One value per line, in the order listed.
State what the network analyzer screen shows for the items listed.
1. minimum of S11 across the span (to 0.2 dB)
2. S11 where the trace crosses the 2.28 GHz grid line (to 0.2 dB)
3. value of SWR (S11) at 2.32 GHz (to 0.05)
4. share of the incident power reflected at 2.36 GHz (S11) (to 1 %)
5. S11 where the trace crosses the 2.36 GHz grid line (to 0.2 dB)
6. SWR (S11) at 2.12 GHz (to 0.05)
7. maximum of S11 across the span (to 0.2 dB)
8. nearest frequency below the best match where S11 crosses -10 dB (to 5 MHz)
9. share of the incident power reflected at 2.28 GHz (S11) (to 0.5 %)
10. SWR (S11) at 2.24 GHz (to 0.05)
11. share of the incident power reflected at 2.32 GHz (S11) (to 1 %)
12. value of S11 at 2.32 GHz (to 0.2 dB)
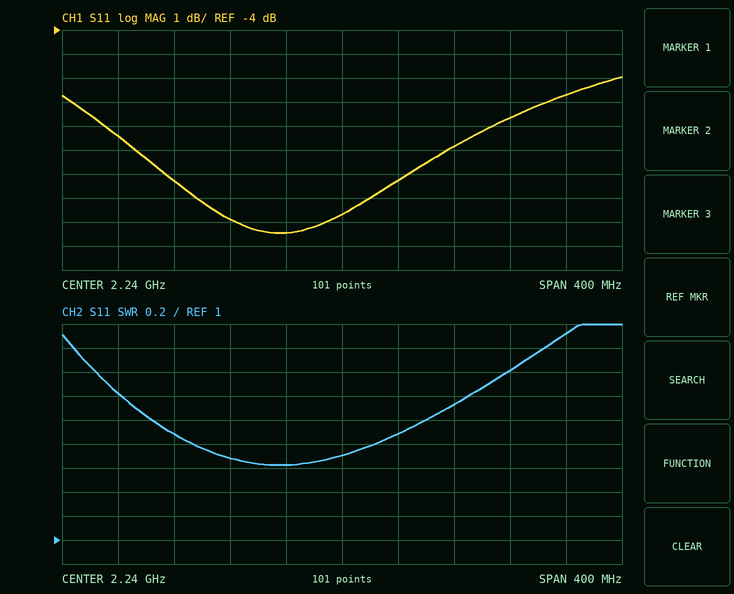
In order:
-12.4 dB
-10.2 dB
2.15
17 %
-7.6 dB
1.90
-6.0 dB
2.115 GHz
9.5 %
1.70
13 %
-8.8 dB
